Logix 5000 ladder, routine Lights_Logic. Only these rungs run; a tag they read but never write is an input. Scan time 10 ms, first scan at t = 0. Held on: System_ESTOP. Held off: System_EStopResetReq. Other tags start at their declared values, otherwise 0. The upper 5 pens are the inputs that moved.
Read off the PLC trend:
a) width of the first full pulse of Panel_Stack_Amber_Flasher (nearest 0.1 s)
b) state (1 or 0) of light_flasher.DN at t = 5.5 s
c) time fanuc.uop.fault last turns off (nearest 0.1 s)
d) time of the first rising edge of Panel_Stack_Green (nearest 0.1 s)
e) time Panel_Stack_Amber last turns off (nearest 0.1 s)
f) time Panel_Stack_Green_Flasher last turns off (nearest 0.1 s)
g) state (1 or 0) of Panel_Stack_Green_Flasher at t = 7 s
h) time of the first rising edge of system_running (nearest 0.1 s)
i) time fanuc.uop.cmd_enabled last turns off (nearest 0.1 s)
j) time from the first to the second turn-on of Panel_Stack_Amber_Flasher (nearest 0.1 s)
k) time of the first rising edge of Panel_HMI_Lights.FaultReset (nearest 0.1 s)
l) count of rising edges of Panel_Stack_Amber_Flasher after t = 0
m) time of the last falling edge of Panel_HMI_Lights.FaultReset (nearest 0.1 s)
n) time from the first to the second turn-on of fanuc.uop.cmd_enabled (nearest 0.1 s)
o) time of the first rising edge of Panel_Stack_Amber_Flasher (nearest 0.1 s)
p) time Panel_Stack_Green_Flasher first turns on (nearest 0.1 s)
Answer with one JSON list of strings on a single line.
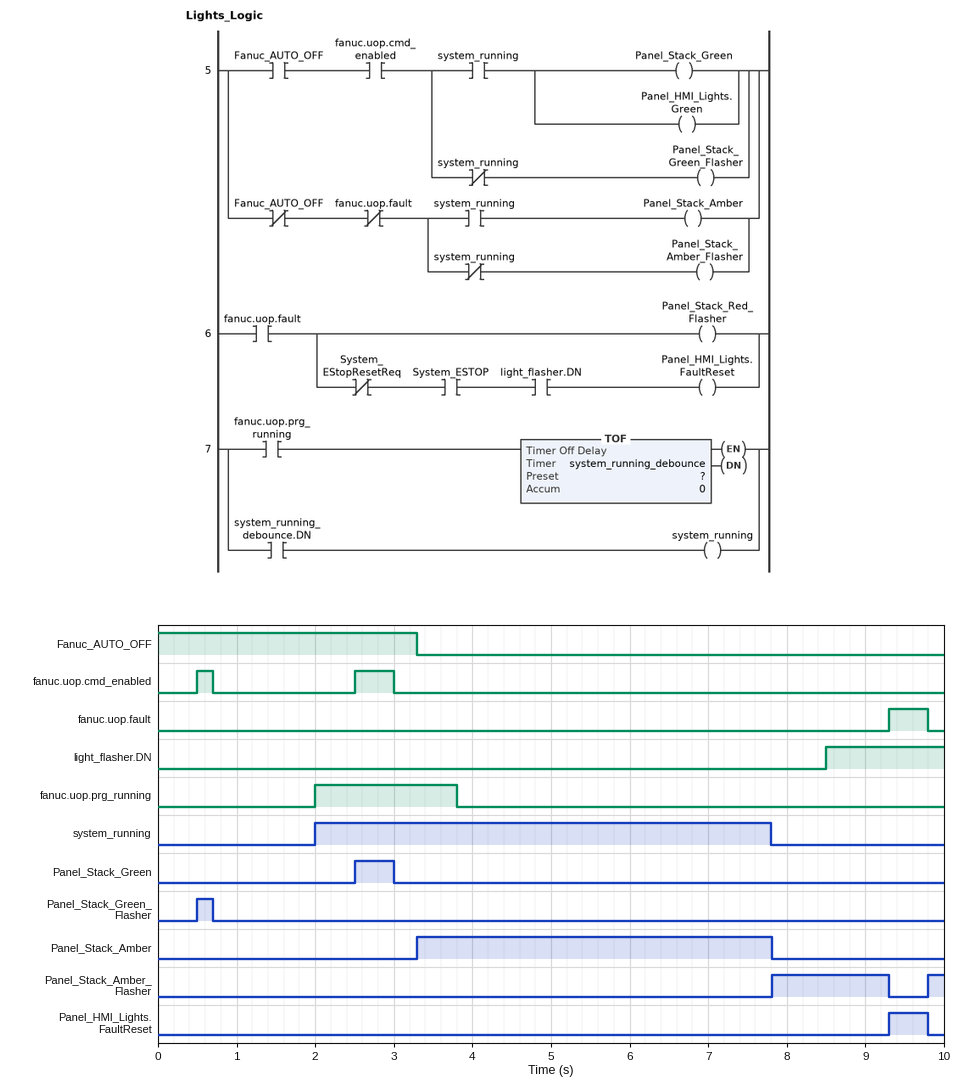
["1.5 s", "0", "9.8 s", "2.5 s", "7.8 s", "0.7 s", "0", "2.0 s", "3.0 s", "2.0 s", "9.3 s", "2", "9.8 s", "2.0 s", "7.8 s", "0.5 s"]
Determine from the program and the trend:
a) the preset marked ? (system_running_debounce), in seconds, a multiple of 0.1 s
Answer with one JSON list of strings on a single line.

["4.0 s"]
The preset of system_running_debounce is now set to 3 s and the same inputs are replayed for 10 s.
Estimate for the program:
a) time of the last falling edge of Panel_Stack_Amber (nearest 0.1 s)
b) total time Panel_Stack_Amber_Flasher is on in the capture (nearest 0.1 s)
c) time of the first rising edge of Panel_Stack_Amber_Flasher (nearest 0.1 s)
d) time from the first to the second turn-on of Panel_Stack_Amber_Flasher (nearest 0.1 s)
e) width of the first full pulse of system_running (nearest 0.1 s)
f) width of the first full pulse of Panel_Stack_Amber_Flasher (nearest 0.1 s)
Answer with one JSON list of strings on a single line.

["6.8 s", "2.7 s", "6.8 s", "3.0 s", "4.8 s", "2.5 s"]
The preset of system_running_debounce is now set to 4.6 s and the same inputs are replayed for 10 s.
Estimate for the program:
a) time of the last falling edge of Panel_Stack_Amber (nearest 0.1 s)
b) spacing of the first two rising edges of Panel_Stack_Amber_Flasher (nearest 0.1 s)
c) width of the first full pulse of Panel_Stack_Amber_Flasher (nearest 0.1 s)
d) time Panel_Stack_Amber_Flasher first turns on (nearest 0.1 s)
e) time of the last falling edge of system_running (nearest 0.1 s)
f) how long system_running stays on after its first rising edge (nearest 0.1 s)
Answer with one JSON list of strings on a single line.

["8.4 s", "1.4 s", "0.9 s", "8.4 s", "8.4 s", "6.4 s"]
